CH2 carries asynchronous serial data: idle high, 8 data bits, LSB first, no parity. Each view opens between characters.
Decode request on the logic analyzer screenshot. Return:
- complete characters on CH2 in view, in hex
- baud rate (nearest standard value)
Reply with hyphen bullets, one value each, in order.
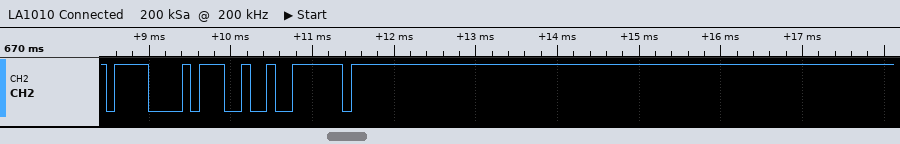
- 0F, 27, 7E
- 9600 baud
